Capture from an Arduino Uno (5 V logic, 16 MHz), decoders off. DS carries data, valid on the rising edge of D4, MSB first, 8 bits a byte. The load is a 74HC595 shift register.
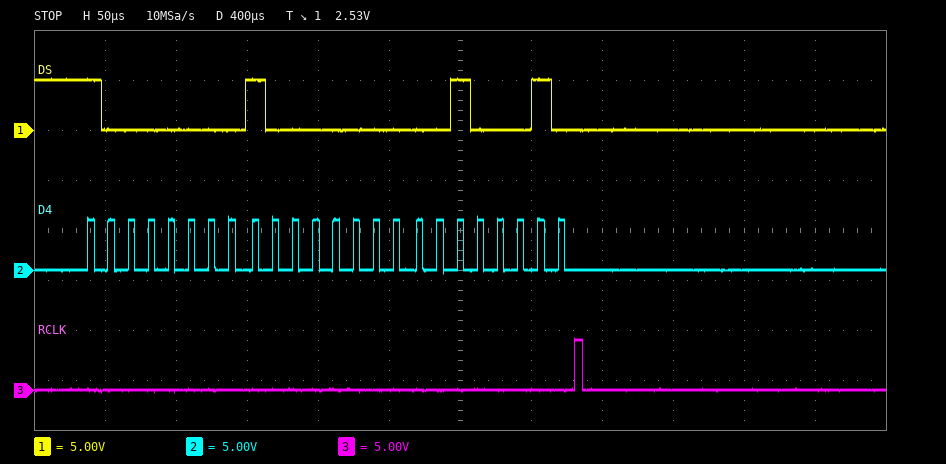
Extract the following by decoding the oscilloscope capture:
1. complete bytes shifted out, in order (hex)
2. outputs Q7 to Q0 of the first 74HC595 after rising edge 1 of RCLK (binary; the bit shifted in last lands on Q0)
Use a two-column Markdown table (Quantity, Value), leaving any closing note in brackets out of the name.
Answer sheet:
| Quantity | Value |
|---|---|
| complete bytes shifted out, in order | 80 80 22 |
| outputs Q7 to Q0 of the first 74HC595 after rising edge 1 of RCLK | 00100010 |
